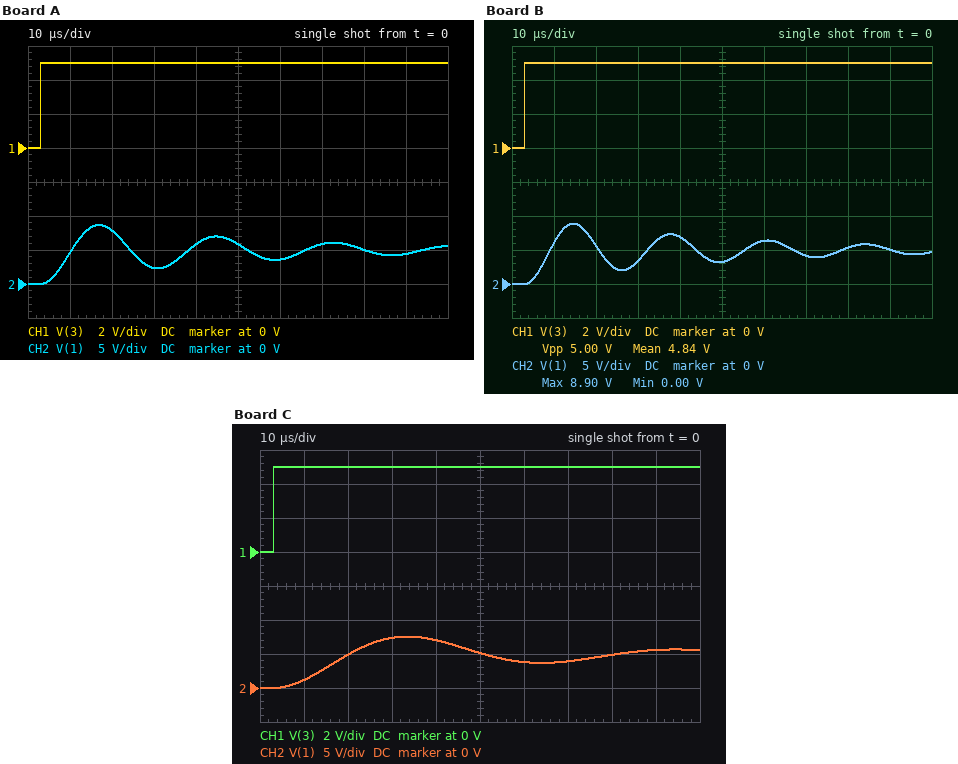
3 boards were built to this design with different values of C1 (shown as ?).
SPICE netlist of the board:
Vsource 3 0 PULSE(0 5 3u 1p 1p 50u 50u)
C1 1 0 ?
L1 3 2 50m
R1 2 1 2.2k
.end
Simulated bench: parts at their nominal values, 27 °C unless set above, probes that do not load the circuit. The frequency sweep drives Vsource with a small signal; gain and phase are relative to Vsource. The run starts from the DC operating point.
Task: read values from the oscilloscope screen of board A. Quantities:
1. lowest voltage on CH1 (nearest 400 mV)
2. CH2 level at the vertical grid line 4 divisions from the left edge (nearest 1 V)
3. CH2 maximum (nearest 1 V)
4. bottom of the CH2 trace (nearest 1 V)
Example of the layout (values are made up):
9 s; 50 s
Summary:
0 V; 6 V; 9 V; 0 V
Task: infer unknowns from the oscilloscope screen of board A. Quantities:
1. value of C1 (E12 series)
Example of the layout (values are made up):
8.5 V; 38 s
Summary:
390 pF
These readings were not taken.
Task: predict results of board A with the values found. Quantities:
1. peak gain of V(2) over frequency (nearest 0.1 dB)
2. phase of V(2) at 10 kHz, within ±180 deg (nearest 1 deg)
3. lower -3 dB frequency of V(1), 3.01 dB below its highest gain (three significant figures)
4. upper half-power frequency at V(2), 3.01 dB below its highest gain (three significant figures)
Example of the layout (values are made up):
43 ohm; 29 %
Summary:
14.4 dB; 0 deg; 32.0 kHz; 39.1 kHz
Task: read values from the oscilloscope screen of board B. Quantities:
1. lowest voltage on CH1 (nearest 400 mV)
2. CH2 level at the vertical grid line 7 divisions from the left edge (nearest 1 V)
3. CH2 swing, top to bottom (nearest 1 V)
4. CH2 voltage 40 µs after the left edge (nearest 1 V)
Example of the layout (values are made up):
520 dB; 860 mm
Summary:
0 V; 4 V; 9 V; 7 V
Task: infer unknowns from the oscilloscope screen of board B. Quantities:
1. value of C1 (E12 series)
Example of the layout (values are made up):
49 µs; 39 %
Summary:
270 pF
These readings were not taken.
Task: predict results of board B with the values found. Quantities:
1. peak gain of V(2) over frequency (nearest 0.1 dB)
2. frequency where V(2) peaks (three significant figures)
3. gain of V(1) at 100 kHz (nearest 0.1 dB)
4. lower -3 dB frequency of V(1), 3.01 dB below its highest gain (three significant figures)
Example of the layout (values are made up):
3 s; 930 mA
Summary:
16.0 dB; 43.0 kHz; -12.8 dB; 39.4 kHz
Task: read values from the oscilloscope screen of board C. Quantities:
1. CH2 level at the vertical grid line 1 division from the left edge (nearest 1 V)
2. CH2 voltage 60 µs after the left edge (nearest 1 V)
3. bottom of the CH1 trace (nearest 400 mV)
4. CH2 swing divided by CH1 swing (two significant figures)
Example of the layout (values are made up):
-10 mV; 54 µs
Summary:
1 V; 4 V; 0 V; 1.5
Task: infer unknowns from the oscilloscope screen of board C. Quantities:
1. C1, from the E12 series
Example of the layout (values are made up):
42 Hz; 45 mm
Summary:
1.8 nF
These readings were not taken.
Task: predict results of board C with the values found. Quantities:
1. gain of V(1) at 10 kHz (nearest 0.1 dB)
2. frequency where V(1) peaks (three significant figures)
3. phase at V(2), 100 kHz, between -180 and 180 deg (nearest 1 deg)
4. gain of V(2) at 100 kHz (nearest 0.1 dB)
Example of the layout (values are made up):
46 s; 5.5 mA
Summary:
3.2 dB; 16.0 kHz; -108 deg; -22.2 dB
